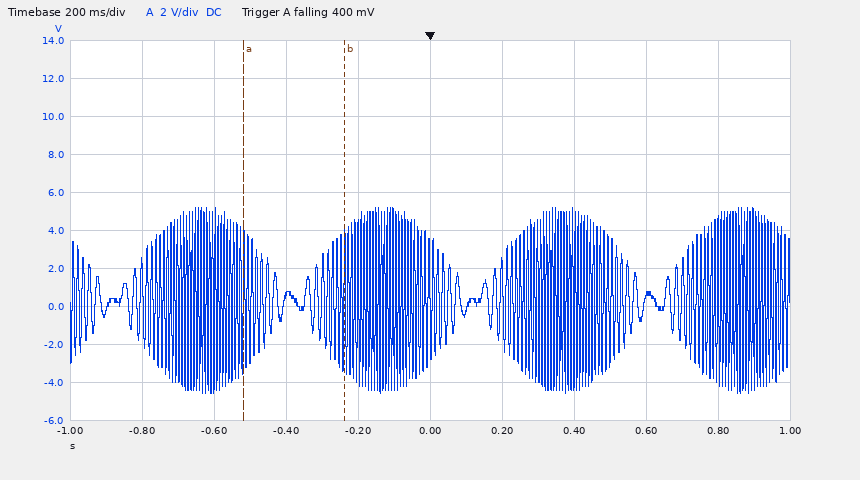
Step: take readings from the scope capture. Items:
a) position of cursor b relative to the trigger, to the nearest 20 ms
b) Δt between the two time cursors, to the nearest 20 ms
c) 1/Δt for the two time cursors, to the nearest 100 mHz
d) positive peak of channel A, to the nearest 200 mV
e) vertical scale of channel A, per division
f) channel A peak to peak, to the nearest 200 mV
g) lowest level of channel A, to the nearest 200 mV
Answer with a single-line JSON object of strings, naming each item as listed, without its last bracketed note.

{"position of cursor b relative to the trigger, to the nearest 20 ms": "-240 ms", "Δt between the two time cursors, to the nearest 20 ms": "280 ms", "1/Δt for the two time cursors, to the nearest 100 mHz": "3.6 Hz", "positive peak of channel A, to the nearest 200 mV": "5.2 V", "vertical scale of channel A, per division": "2 V", "channel A peak to peak, to the nearest 200 mV": "9.8 V", "lowest level of channel A, to the nearest 200 mV": "-4.6 V"}
